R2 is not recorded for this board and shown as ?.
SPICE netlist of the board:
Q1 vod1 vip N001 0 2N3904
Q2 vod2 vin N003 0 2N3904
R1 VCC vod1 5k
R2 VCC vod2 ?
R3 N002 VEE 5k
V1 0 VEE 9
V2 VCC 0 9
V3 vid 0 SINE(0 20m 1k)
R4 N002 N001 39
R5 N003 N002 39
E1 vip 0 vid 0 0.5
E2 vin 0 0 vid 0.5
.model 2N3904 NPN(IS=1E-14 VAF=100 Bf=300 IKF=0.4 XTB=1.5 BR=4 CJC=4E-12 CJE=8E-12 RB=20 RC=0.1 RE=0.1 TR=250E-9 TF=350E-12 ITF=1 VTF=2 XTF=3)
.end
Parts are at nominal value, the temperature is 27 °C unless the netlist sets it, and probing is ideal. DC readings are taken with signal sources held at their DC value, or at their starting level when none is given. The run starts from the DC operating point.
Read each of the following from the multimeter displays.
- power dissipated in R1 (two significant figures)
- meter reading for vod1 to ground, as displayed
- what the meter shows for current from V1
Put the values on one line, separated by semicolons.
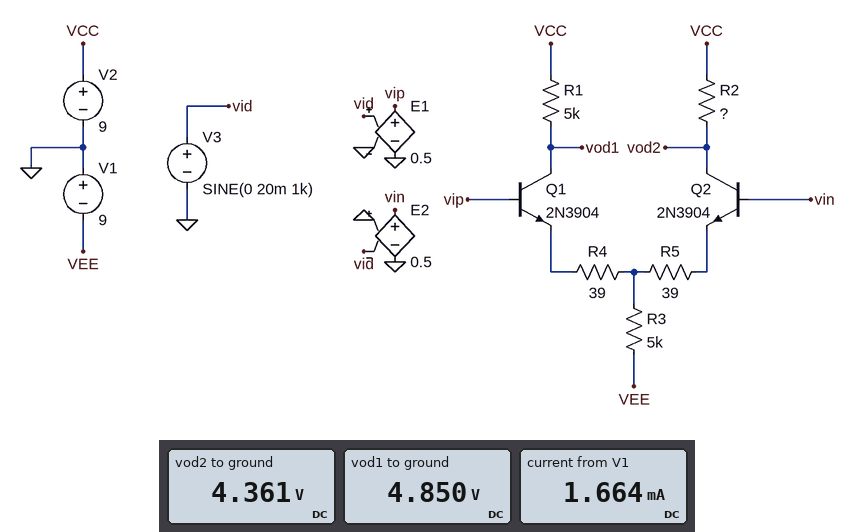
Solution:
3.4 mW; 4.850 V; 1.664 mA
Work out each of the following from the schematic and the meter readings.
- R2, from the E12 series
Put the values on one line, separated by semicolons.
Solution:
5.6 kΩ
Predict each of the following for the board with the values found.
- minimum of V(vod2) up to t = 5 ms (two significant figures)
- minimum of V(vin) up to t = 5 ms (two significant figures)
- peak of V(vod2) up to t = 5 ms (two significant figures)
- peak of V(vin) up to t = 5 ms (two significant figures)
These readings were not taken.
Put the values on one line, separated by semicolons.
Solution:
3.6 V; -10 mV; 5.1 V; 10 mV
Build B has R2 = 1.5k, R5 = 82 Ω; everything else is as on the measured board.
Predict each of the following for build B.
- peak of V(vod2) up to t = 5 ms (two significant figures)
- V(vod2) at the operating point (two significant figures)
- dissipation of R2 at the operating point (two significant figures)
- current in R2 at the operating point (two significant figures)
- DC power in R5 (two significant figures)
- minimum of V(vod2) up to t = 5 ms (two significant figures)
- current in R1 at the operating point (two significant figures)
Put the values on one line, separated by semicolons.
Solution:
8.2 V; 8.0 V; 620 µW; 640 µA; 34 µW; 7.9 V; 1.0 mA
